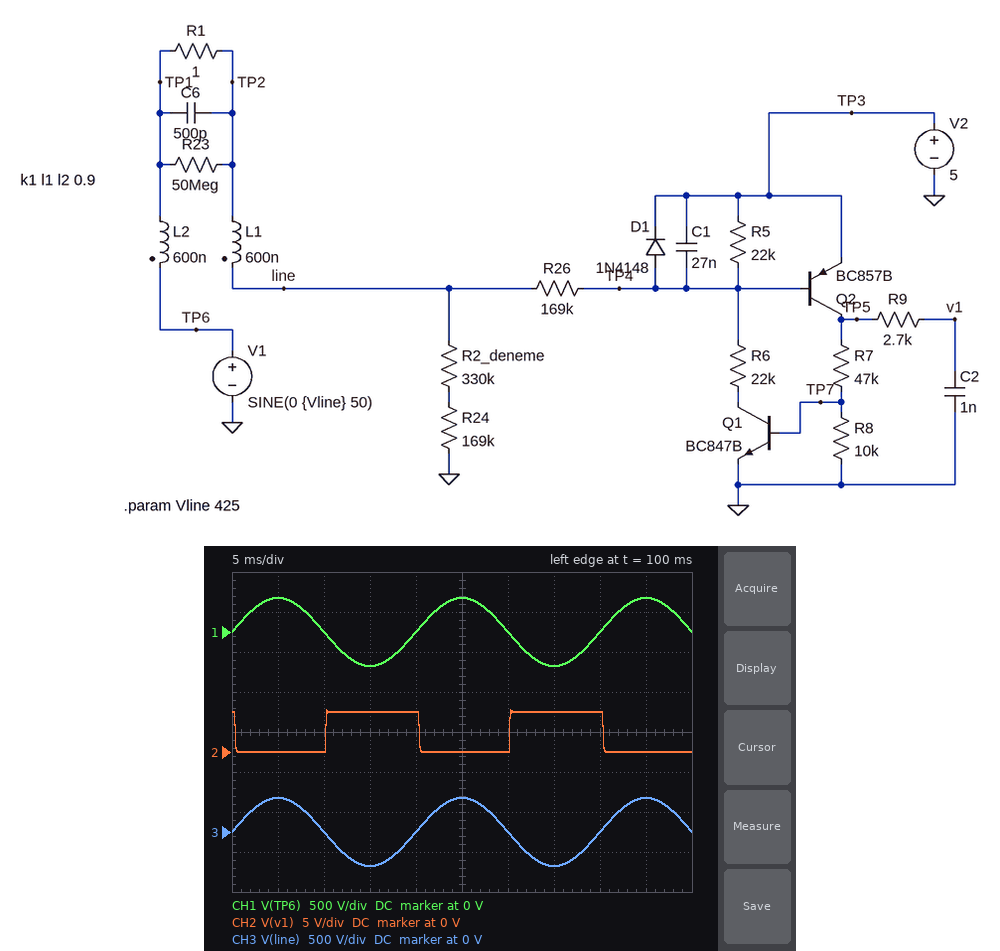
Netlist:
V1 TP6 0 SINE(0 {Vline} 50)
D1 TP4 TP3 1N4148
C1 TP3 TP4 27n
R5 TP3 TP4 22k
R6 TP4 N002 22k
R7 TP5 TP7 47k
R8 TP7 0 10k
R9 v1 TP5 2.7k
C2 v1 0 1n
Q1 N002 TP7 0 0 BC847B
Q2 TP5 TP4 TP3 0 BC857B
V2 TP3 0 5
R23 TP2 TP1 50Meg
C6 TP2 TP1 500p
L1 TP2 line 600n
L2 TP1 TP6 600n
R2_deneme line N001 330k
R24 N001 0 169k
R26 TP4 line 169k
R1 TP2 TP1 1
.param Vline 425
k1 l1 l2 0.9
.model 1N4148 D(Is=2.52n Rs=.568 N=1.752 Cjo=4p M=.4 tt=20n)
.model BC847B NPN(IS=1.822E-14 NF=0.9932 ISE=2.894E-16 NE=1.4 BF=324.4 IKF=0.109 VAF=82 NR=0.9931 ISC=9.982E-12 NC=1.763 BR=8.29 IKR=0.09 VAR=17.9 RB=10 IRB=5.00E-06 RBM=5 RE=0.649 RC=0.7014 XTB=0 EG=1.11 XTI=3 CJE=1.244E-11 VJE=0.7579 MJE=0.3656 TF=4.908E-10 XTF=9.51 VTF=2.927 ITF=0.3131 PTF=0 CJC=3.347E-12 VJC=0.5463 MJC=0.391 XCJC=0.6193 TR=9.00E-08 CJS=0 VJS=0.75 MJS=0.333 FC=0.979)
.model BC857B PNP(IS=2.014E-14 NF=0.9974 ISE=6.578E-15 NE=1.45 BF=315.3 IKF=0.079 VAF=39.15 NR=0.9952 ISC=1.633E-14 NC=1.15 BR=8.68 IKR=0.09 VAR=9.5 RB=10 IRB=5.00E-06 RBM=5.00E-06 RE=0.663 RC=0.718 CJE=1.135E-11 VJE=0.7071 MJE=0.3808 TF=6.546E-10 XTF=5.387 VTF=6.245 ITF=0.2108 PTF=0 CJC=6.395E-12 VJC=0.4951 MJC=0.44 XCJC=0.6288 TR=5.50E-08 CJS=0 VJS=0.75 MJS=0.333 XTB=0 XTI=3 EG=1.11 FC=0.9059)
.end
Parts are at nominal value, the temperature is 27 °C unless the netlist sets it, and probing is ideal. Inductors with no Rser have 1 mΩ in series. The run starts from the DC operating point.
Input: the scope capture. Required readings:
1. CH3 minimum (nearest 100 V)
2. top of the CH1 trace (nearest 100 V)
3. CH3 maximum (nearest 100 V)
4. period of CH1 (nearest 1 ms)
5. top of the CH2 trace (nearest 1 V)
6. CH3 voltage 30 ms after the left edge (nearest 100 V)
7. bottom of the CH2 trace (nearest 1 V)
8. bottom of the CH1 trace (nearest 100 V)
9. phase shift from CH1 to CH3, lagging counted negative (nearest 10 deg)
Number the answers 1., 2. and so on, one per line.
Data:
1. -400 V
2. 400 V
3. 400 V
4. 20 ms
5. 5 V
6. 0 V
7. 0 V
8. -400 V
9. 0 deg
